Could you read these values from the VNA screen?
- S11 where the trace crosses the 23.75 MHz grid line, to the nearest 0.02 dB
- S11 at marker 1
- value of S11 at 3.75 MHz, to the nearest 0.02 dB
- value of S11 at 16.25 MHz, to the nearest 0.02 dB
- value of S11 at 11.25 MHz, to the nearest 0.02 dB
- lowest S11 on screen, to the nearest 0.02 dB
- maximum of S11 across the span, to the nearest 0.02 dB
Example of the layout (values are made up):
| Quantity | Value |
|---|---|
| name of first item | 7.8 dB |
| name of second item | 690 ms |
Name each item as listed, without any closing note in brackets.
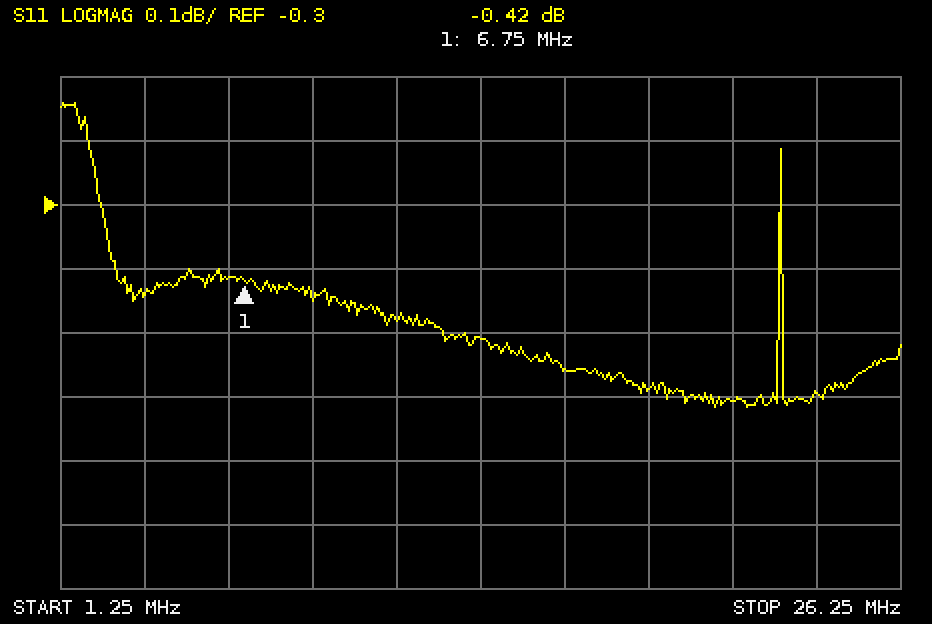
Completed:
| Quantity | Value |
|---|---|
| S11 where the trace crosses the 23.75 MHz grid line, to the nearest 0.02 dB | -0.60 dB |
| S11 at marker 1 | -0.42 dB |
| value of S11 at 3.75 MHz, to the nearest 0.02 dB | -0.44 dB |
| value of S11 at 16.25 MHz, to the nearest 0.02 dB | -0.56 dB |
| value of S11 at 11.25 MHz, to the nearest 0.02 dB | -0.48 dB |
| lowest S11 on screen, to the nearest 0.02 dB | -0.62 dB |
| maximum of S11 across the span, to the nearest 0.02 dB | -0.14 dB |
